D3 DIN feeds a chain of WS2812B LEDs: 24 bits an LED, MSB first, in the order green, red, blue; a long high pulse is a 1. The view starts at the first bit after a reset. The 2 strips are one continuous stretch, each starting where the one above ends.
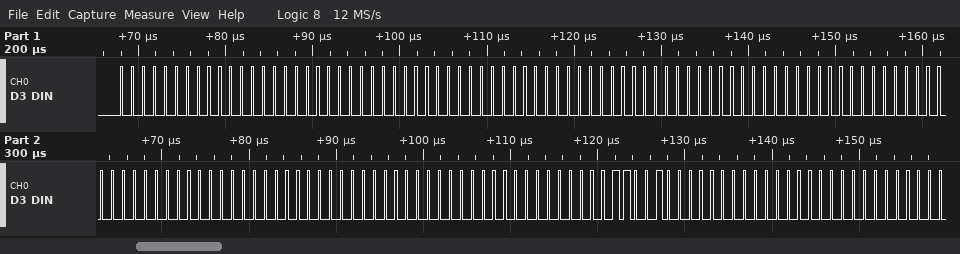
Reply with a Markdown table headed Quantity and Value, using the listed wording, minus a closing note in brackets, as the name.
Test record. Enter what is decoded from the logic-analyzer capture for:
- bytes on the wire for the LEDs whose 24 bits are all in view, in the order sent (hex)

| Quantity | Value |
|---|---|
| bytes on the wire for the LEDs whose 24 bits are all in view, in the order sent | 00 00 00 00 00 00 00 00 00 00 00 00 00 00 00 19 00 00 |
